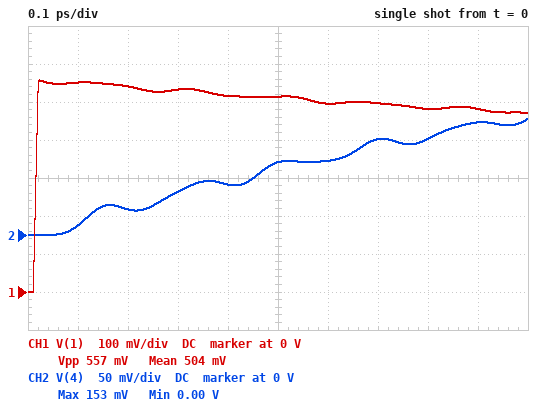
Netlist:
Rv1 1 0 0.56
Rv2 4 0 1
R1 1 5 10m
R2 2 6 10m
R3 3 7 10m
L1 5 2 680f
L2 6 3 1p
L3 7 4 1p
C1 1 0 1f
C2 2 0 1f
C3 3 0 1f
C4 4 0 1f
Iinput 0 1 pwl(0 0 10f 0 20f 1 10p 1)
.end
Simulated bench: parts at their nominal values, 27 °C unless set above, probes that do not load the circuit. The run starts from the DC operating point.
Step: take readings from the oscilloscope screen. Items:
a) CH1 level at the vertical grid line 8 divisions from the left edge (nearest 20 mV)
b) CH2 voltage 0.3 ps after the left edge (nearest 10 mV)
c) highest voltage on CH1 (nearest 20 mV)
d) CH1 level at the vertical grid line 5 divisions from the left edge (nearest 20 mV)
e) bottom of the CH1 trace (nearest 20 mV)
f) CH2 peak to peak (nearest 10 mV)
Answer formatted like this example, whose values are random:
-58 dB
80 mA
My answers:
480 mV
60 mV
560 mV
520 mV
0 V
150 mV
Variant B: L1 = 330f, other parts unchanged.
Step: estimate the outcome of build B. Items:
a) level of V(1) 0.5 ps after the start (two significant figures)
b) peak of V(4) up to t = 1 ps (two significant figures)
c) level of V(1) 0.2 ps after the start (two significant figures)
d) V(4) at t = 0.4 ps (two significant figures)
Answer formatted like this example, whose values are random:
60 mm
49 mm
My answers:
500 mV
170 mV
530 mV
79 mV
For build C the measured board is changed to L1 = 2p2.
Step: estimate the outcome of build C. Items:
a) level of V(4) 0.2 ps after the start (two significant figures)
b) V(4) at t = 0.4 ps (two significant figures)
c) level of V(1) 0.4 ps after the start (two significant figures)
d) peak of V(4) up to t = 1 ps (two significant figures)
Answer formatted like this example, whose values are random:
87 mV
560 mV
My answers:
30 mV
52 mV
530 mV
110 mV
